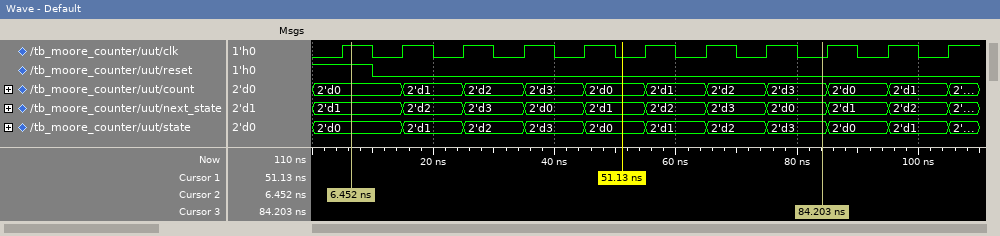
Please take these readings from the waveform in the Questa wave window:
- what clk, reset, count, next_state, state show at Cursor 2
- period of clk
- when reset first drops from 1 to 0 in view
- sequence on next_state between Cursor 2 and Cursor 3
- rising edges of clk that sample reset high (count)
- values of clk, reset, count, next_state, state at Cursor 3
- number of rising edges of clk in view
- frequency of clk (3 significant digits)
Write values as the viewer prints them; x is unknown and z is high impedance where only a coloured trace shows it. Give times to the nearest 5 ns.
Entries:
clk=1, reset=1, count=2'd0, next_state=2'd1, state=2'd0
10 ns
10 ns
2'd1, 2'd2, 2'd3, 2'd0, 2'd1, 2'd2, 2'd3, 2'd0
1
clk=0, reset=0, count=2'd3, next_state=2'd0, state=2'd3
11
100 MHz
